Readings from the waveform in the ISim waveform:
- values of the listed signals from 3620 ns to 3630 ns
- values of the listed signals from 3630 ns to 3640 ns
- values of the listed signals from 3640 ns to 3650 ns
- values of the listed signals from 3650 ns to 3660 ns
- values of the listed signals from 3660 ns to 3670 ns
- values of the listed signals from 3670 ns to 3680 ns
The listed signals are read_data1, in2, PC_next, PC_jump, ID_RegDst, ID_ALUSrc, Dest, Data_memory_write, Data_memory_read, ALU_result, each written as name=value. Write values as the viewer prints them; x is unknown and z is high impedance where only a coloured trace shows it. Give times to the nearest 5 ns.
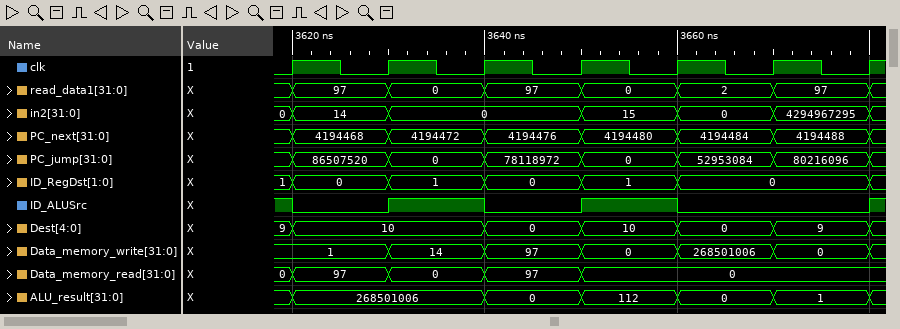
read_data1=97, in2=14, PC_next=4194468, PC_jump=86507520, ID_RegDst=0, ID_ALUSrc=0, Dest=10, Data_memory_write=1, Data_memory_read=97, ALU_result=268501006
read_data1=0, in2=0, PC_next=4194472, PC_jump=0, ID_RegDst=1, ID_ALUSrc=1, Dest=10, Data_memory_write=14, Data_memory_read=0, ALU_result=268501006
read_data1=97, in2=0, PC_next=4194476, PC_jump=78118972, ID_RegDst=0, ID_ALUSrc=0, Dest=0, Data_memory_write=97, Data_memory_read=97, ALU_result=0
read_data1=0, in2=15, PC_next=4194480, PC_jump=0, ID_RegDst=1, ID_ALUSrc=1, Dest=10, Data_memory_write=0, Data_memory_read=0, ALU_result=112
read_data1=2, in2=0, PC_next=4194484, PC_jump=52953084, ID_RegDst=0, ID_ALUSrc=0, Dest=0, Data_memory_write=268501006, Data_memory_read=0, ALU_result=0
read_data1=97, in2=4294967295, PC_next=4194488, PC_jump=80216096, ID_RegDst=0, ID_ALUSrc=0, Dest=9, Data_memory_write=0, Data_memory_read=0, ALU_result=1
